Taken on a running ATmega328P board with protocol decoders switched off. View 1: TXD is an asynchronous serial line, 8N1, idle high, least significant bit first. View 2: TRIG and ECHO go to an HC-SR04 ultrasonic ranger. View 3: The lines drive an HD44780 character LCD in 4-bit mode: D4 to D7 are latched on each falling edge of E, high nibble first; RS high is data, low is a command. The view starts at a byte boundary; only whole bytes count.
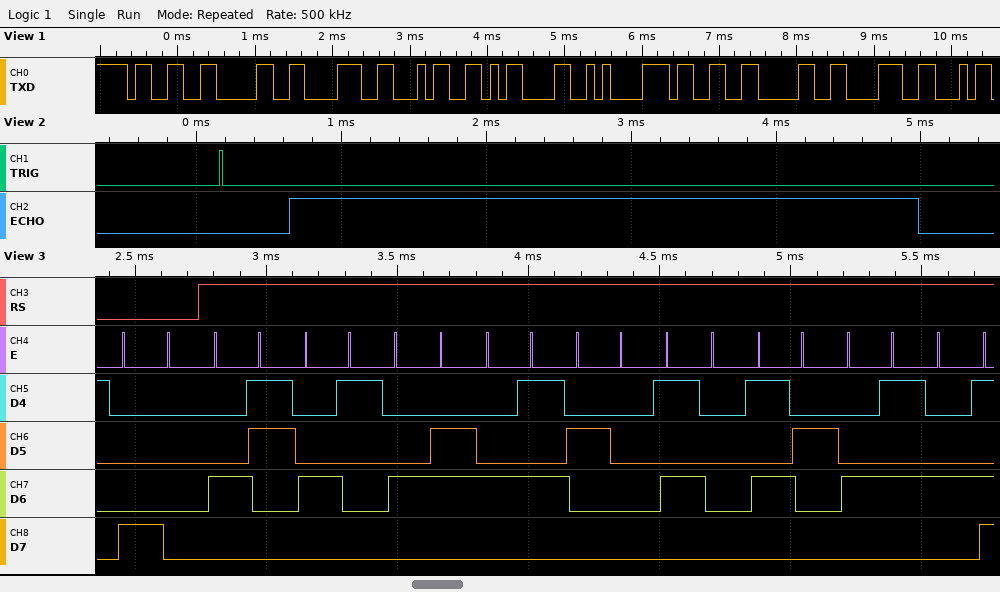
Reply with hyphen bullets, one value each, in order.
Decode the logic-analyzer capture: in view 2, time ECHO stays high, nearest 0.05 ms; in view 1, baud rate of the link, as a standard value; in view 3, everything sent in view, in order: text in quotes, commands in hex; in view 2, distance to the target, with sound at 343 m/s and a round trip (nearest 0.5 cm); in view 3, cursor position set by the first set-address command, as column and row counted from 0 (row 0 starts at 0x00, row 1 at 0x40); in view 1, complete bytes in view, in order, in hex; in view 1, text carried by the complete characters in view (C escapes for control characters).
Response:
- 4.35 ms
- 9600 baud
- 0x80 "CAFE PREM"
- 74.5 cm
- column 0, row 0
- 33 30 38 34 0D 0A 33 30 38
- "3084\r\n308"
